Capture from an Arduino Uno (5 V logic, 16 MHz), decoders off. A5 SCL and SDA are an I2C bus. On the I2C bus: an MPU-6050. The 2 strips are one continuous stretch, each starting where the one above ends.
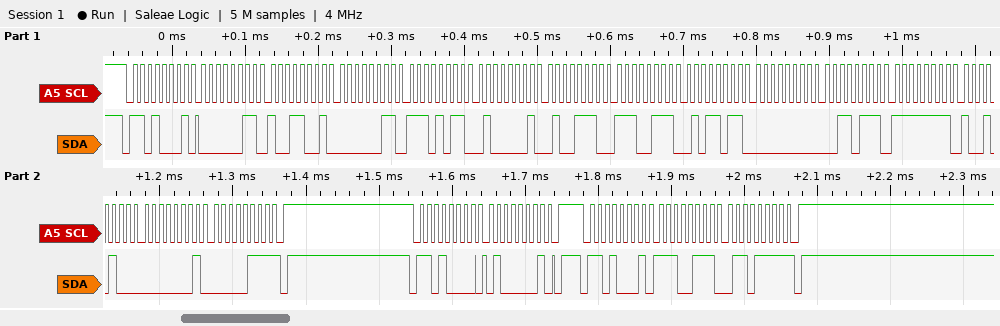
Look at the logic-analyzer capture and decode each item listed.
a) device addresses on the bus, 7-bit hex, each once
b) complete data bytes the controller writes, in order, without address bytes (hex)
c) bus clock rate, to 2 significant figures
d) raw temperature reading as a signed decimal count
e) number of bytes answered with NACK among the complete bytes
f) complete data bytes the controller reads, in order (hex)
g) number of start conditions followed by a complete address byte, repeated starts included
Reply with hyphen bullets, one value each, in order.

- 0x68
- 41
- 100 kHz
- -6289
- 2
- 03 99 03 EB 41 4E E7 5B 00 37 FF 94 01 07 E7 6F
- 3
